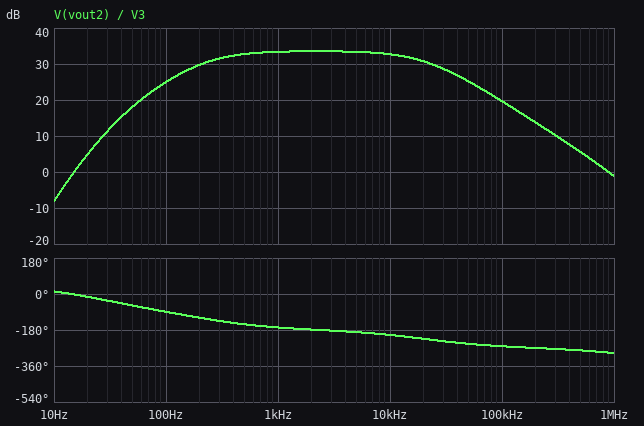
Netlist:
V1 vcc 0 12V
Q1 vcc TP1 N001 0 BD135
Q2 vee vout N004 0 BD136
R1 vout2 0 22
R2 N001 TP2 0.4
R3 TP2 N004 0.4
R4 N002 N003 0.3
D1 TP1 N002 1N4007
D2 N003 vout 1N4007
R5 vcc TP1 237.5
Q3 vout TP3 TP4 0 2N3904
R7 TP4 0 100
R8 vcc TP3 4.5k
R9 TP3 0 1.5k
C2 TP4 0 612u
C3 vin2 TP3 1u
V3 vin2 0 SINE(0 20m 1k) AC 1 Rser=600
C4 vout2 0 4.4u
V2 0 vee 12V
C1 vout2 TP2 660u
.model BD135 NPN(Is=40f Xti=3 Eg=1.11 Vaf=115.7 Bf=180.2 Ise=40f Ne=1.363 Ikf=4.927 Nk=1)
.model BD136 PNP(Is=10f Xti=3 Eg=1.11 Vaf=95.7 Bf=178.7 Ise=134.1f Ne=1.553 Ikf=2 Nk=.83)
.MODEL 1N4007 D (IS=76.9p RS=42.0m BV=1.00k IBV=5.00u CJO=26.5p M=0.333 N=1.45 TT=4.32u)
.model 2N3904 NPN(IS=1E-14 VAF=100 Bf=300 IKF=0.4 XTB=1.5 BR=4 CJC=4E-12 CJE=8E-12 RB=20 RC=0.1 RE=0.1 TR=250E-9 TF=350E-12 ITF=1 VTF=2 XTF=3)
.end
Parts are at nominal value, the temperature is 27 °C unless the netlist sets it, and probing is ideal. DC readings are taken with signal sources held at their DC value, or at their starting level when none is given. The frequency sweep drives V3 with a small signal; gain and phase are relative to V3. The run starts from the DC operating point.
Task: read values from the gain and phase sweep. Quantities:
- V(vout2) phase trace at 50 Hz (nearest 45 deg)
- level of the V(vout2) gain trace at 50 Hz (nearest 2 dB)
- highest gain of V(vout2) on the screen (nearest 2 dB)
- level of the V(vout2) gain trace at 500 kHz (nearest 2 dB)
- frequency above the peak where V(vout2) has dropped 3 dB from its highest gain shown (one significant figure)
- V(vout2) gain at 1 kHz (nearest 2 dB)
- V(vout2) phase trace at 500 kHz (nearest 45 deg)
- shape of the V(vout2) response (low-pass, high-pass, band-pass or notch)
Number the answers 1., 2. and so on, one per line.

1. -45 deg
2. 18 dB
3. 34 dB
4. 6 dB
5. 20 kHz
6. 34 dB
7. -270 deg
8. band-pass
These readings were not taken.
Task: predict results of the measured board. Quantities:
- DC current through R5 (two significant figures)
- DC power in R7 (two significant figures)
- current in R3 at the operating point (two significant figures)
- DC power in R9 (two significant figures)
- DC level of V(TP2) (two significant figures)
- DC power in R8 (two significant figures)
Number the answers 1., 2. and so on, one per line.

1. 22 mA
2. 47 mW
3. 29 mA
4. 5.7 mW
5. 6.1 V
6. 18 mW
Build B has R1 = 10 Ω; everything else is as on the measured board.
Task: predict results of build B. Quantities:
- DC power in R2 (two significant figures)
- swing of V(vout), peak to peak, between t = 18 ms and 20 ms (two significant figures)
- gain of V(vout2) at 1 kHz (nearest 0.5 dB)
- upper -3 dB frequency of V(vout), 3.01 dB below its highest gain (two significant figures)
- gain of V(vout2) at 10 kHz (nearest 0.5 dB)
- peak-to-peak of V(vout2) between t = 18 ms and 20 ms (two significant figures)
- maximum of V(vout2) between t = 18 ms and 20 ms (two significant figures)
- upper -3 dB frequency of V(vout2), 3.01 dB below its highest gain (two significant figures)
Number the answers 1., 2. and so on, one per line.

1. 340 µW
2. 1.8 V
3. 32.5 dB
4. 27 kHz
5. 32.0 dB
6. 1.7 V
7. 830 mV
8. 23 kHz
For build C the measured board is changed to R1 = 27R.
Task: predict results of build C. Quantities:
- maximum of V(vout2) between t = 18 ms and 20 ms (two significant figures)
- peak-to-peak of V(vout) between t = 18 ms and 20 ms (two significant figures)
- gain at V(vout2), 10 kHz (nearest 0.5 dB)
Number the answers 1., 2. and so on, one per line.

1. 930 mV
2. 2.0 V
3. 33.0 dB
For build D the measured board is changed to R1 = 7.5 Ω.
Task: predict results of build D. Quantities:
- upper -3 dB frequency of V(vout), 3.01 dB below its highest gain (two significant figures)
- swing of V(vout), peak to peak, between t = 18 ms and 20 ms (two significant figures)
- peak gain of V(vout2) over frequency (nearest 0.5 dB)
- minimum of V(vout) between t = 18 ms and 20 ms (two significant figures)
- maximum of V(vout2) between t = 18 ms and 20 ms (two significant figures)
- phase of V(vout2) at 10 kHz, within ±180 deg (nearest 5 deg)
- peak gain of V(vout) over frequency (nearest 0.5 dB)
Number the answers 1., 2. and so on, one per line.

1. 29 kHz
2. 1.8 V
3. 32.5 dB
4. 4.5 V
5. 790 mV
6. 160 deg
7. 33.0 dB
